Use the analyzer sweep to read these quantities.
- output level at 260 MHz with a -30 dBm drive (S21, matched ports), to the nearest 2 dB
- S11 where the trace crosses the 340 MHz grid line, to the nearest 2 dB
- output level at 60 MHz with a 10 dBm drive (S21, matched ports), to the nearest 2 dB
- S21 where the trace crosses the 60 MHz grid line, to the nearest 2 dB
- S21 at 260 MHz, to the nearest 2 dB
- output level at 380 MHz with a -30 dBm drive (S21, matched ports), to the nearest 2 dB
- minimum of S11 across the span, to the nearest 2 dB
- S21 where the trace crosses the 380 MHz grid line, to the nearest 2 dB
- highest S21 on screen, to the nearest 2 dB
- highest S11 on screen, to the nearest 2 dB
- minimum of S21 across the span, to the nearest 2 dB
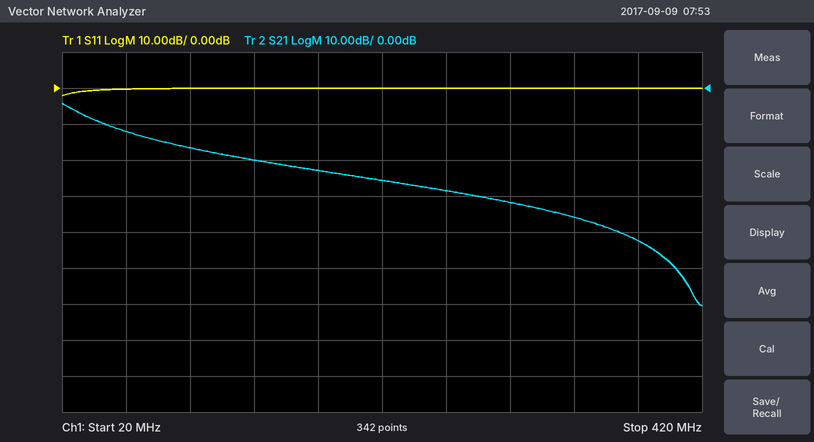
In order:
-58 dBm
0 dB
-2 dBm
-12 dB
-28 dB
-72 dBm
-2 dB
-42 dB
-4 dB
0 dB
-60 dB
